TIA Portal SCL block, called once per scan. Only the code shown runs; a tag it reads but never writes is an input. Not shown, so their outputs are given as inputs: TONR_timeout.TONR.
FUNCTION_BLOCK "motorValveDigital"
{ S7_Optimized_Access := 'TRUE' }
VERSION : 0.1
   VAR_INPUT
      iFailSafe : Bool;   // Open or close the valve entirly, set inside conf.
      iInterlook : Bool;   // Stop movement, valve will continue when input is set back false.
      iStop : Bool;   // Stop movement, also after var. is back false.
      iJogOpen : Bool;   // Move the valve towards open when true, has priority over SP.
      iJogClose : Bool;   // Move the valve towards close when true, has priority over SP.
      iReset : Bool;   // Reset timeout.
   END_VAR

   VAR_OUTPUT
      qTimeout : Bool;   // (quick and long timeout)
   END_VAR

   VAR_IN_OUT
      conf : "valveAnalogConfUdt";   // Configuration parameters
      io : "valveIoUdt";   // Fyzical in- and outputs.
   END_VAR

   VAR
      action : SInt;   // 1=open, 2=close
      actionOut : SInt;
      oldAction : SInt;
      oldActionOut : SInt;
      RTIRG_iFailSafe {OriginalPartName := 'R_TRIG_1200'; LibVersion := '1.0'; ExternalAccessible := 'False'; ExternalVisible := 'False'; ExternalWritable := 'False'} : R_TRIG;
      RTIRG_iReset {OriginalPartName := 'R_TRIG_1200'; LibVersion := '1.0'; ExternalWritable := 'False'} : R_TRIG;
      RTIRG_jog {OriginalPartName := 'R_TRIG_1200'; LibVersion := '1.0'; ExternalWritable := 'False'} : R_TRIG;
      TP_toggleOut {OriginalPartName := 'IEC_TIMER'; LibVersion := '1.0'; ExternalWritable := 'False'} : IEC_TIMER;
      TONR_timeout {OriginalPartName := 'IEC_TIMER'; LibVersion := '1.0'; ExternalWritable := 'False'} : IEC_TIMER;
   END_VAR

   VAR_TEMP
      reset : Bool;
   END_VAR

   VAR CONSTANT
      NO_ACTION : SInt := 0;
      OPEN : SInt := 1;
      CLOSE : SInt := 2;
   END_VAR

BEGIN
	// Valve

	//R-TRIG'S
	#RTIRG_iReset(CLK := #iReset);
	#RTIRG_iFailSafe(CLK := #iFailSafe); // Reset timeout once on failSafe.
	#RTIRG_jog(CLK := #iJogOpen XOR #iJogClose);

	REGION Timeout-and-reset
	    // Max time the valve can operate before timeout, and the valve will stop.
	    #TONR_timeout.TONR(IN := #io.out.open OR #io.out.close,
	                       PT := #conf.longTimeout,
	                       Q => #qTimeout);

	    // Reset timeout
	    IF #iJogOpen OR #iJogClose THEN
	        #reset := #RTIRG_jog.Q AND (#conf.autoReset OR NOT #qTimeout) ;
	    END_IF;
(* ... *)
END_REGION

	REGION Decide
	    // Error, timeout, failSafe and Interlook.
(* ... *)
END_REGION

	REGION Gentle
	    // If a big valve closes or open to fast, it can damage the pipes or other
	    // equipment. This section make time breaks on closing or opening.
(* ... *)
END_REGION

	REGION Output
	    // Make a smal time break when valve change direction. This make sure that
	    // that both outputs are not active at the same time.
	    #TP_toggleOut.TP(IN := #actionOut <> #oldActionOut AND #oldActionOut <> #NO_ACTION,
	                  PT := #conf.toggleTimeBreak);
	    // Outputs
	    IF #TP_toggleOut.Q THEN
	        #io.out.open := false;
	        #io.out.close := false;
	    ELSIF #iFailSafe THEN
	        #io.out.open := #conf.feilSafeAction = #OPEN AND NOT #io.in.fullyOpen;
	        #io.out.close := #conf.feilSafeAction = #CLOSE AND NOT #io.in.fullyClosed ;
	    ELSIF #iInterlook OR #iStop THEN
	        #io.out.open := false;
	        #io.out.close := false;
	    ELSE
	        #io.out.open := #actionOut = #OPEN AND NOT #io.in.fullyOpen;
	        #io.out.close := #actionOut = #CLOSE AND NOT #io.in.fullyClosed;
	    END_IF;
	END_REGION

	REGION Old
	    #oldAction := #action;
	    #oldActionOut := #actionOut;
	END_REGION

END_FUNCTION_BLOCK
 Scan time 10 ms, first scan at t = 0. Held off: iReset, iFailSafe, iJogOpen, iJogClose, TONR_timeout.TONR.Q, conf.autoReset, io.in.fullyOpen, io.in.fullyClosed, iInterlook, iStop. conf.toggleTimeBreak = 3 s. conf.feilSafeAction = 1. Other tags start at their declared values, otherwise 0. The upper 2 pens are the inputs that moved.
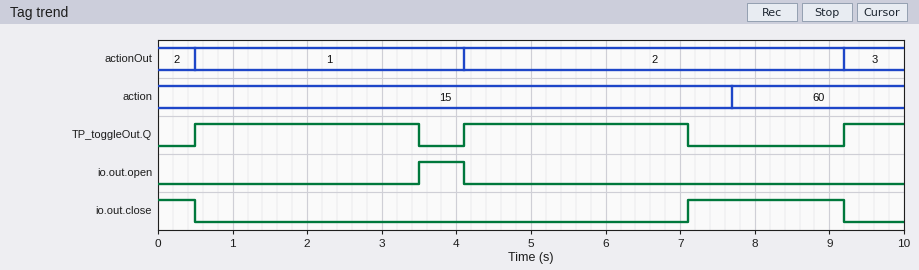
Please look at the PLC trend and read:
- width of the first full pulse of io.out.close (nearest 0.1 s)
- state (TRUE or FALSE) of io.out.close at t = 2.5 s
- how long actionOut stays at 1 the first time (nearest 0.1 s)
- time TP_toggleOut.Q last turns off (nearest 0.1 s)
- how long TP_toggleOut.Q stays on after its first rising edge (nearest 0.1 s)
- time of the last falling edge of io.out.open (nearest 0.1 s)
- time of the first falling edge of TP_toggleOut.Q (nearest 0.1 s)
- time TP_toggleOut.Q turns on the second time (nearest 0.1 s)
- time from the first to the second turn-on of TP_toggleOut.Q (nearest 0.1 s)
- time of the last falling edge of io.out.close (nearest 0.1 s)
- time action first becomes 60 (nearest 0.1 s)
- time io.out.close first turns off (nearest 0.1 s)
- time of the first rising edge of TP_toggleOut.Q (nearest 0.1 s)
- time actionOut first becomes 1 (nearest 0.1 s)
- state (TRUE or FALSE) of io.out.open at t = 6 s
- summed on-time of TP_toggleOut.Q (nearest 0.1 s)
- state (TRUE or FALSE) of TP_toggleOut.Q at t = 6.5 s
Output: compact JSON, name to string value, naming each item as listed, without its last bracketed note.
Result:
{"width of the first full pulse of io.out.close": "2.1 s", "state (TRUE or FALSE) of io.out.close at t = 2.5 s": "FALSE", "how long actionOut stays at 1 the first time": "3.6 s", "time TP_toggleOut.Q last turns off": "7.1 s", "how long TP_toggleOut.Q stays on after its first rising edge": "3.0 s", "time of the last falling edge of io.out.open": "4.1 s", "time of the first falling edge of TP_toggleOut.Q": "3.5 s", "time TP_toggleOut.Q turns on the second time": "4.1 s", "time from the first to the second turn-on of TP_toggleOut.Q": "3.6 s", "time of the last falling edge of io.out.close": "9.2 s", "time action first becomes 60": "7.7 s", "time io.out.close first turns off": "0.5 s", "time of the first rising edge of TP_toggleOut.Q": "0.5 s", "time actionOut first becomes 1": "0.5 s", "state (TRUE or FALSE) of io.out.open at t = 6 s": "FALSE", "summed on-time of TP_toggleOut.Q": "6.8 s", "state (TRUE or FALSE) of TP_toggleOut.Q at t = 6.5 s": "TRUE"}
